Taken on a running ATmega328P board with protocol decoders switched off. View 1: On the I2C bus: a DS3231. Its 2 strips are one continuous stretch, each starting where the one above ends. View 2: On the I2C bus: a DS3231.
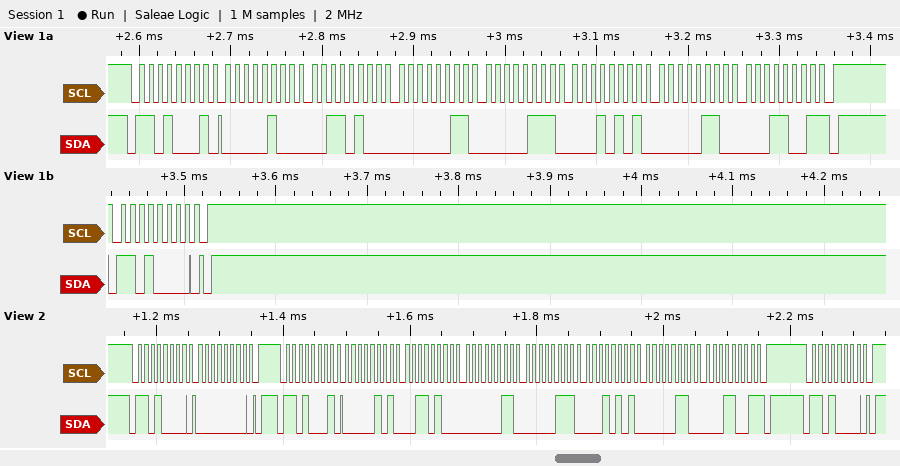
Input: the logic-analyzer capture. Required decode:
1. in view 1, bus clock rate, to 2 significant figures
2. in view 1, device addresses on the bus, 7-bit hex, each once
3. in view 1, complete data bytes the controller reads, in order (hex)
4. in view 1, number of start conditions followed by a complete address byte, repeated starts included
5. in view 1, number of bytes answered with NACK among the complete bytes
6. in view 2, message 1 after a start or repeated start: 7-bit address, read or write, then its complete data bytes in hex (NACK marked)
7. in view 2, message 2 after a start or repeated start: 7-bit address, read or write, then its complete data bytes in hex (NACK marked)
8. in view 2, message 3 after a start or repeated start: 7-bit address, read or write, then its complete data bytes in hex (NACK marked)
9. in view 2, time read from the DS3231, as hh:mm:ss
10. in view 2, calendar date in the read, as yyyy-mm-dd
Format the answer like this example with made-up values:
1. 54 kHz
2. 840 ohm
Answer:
1. 100 kHz
2. 0x68
3. 04 34 03 07 15 06 19
4. 2
5. 1
6. 0x68 write: 00
7. 0x68 read: 05 34 03 07 15 06 19 NACK
8. 0x68 write
9. 03:34:05
10. 2019-06-15
